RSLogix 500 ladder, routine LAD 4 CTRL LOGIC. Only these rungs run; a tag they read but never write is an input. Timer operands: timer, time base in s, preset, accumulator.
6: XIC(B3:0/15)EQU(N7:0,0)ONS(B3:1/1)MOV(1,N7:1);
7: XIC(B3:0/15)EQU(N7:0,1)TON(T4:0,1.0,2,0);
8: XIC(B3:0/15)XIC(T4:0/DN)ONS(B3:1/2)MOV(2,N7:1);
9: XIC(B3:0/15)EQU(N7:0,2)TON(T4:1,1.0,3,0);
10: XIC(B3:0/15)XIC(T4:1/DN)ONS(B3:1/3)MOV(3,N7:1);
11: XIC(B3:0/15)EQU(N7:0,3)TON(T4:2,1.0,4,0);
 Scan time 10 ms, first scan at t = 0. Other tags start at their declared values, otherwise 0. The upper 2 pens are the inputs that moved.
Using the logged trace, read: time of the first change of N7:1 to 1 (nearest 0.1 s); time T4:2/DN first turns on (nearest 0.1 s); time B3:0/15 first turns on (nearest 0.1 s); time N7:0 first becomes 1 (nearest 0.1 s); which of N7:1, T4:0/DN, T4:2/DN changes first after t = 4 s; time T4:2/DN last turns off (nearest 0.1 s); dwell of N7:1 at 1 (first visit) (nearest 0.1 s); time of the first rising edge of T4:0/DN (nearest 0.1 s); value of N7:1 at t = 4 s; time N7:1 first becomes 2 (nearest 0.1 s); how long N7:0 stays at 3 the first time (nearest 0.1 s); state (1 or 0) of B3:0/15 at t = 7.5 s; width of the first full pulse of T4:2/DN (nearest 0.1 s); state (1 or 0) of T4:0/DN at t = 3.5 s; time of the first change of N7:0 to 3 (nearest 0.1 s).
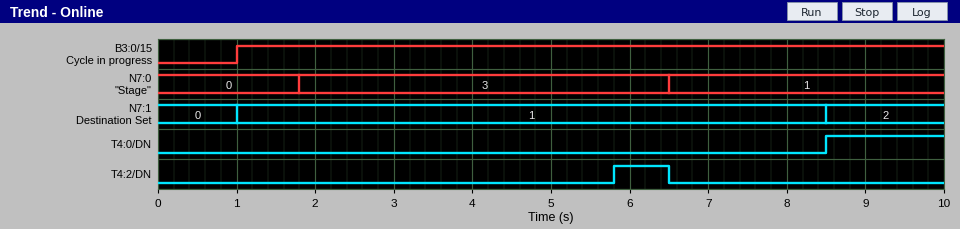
1.0 s
5.8 s
1.0 s
6.5 s
T4:2/DN
6.5 s
7.5 s
8.5 s
1
8.5 s
4.7 s
1
0.7 s
0
1.8 s
